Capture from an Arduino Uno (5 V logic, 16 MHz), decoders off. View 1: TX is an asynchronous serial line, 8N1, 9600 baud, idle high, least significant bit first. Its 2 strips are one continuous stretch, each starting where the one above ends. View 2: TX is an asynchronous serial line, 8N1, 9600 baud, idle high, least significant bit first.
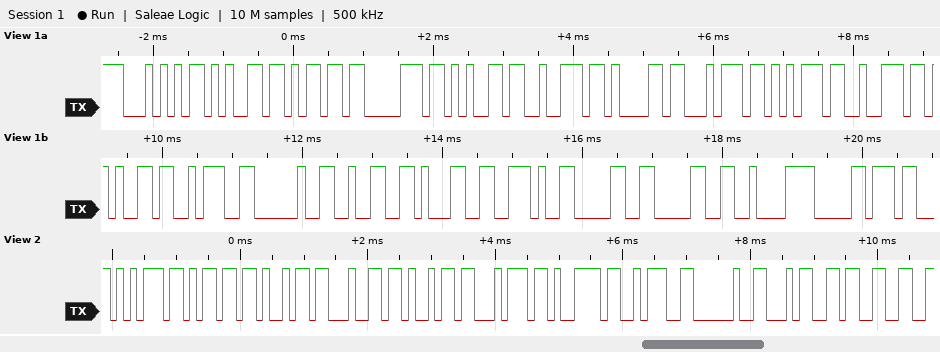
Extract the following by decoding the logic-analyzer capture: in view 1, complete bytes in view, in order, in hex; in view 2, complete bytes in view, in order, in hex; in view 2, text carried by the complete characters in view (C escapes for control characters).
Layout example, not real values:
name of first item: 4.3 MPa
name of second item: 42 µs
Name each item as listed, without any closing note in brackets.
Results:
in view 1, complete bytes in view, in order, in hex: 54 65 6D 70 65 72 61 74 75 72 65 3A 20 32 31 2E 30 30 C2 B0
in view 2, complete bytes in view, in order, in hex: 75 6D 69 64 69 74 79 3A 20 34 33
in view 2, text carried by the complete characters in view: "umidity: 43"
